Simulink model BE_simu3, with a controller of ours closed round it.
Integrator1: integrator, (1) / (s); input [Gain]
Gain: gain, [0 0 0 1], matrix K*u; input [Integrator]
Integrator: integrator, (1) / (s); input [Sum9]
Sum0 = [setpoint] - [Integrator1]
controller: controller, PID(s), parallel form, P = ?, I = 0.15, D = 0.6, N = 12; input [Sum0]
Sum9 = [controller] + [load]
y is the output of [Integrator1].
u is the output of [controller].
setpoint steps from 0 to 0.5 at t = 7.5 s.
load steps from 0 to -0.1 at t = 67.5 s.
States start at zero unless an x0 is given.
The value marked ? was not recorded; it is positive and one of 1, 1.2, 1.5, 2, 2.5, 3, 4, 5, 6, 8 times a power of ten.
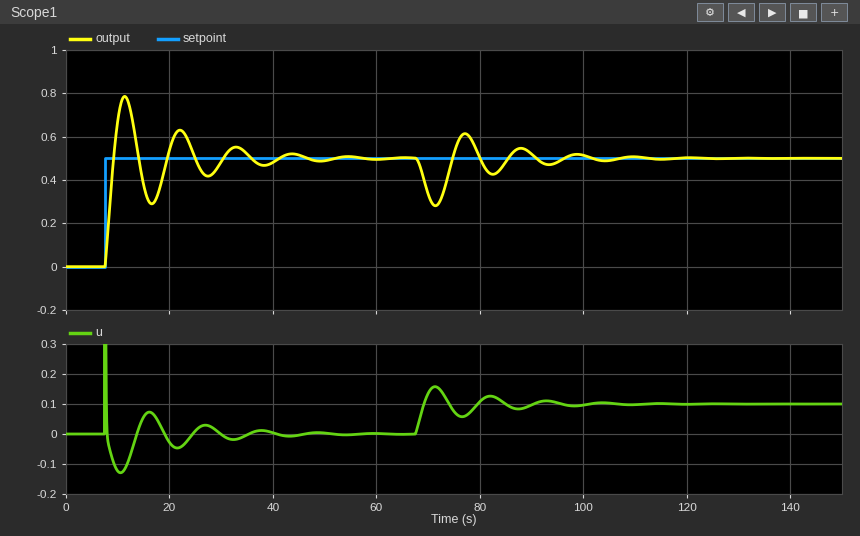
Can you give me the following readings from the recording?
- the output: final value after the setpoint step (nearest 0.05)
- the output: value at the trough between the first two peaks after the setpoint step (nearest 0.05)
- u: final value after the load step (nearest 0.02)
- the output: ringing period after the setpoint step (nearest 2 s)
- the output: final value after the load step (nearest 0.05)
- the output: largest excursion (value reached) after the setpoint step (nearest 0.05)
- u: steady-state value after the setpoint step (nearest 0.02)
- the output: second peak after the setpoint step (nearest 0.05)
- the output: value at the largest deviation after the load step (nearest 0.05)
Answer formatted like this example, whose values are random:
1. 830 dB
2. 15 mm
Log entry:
1. 0.50
2. 0.30
3. 0.10
4. 10 s
5. 0.50
6. 0.80
7. 0.00
8. 0.65
9. 0.30
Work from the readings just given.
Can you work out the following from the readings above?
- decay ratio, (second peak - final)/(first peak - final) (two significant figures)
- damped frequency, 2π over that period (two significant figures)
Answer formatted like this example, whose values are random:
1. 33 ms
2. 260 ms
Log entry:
1. 0.50
2. 0.63 rad/s
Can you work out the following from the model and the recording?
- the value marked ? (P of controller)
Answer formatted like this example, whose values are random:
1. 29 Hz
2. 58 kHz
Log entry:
1. 0.4
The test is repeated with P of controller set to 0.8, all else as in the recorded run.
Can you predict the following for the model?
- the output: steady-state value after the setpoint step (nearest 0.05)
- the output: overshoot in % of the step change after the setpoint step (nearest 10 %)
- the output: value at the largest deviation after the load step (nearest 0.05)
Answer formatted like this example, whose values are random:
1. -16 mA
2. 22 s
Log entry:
1. 0.50
2. 60 %
3. 0.35
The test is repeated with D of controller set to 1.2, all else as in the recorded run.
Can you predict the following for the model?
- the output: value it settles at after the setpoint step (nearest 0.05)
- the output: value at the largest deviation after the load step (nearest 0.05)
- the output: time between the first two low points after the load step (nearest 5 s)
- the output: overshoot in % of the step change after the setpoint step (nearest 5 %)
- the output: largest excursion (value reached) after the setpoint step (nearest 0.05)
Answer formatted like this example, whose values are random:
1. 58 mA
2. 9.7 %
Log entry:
1. 0.50
2. 0.35
3. 15 s
4. 25 %
5. 0.65
